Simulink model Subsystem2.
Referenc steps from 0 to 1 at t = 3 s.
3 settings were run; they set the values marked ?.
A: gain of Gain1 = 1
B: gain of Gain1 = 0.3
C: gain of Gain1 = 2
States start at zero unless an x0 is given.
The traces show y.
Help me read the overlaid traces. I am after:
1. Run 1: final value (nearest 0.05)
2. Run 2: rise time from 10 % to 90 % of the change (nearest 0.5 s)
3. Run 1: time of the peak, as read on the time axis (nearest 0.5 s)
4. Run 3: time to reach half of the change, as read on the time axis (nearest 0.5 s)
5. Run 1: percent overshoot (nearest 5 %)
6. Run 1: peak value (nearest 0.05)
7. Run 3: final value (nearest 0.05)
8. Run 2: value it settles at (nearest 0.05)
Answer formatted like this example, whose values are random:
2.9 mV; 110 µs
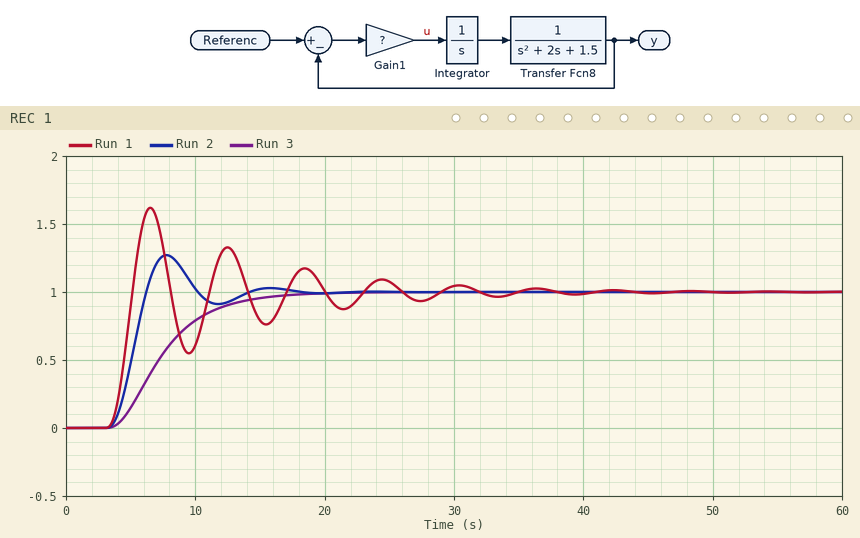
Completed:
1.00; 2.0 s; 6.5 s; 7.0 s; 60 %; 1.60; 1.00; 1.00
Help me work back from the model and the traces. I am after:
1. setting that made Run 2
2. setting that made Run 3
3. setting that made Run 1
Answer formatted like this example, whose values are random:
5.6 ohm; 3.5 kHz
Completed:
A; B; C
